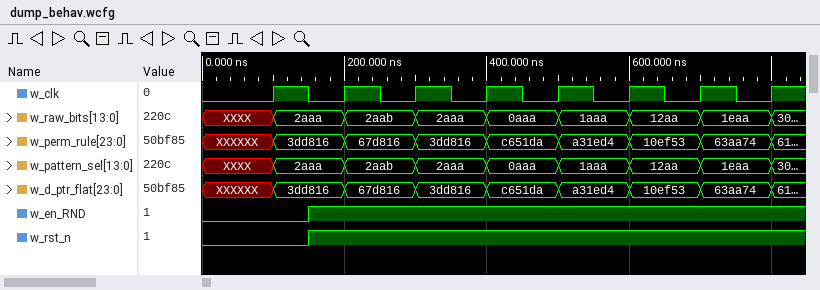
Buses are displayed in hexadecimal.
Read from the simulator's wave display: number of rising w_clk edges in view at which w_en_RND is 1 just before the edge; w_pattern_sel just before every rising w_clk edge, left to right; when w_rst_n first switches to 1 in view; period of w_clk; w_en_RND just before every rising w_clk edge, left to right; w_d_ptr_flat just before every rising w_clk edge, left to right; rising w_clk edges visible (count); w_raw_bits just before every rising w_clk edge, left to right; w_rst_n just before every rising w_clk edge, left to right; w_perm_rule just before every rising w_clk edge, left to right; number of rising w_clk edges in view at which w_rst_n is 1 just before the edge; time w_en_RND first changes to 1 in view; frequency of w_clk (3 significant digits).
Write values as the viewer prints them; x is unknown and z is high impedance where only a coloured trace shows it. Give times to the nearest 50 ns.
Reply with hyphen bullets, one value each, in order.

- 7
- XXXX, 2aaa, 2aab, 2aaa, 0aaa, 1aaa, 12aa, 1eaa
- 150 ns
- 100 ns
- 0 1 1 1 1 1 1 1
- XXXXXX, 3dd816, 67d816, 3dd816, c651da, a31ed4, 10ef53, 63aa74
- 8
- XXXX, 2aaa, 2aab, 2aaa, 0aaa, 1aaa, 12aa, 1eaa
- 0 1 1 1 1 1 1 1
- XXXXXX, 3dd816, 67d816, 3dd816, c651da, a31ed4, 10ef53, 63aa74
- 7
- 150 ns
- 10.0 MHz
